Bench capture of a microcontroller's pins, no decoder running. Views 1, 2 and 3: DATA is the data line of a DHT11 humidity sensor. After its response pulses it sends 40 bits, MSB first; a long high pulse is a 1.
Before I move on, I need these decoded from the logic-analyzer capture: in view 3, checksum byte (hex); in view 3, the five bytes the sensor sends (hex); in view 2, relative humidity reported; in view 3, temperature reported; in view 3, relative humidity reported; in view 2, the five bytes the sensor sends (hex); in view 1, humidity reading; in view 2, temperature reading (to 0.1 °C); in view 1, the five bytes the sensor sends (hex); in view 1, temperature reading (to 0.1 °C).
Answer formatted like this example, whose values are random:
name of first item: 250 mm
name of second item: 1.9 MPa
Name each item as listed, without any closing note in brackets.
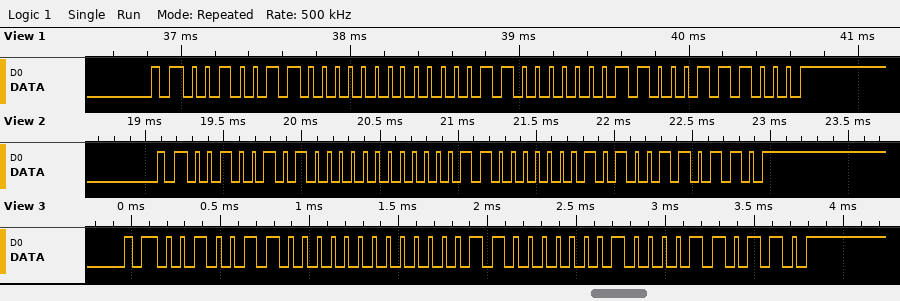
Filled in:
in view 3, checksum byte: 0x36
in view 3, the five bytes the sensor sends: 26 00 0C 04 36
in view 2, relative humidity reported: 37 %
in view 3, temperature reported: 12.4 °C
in view 3, relative humidity reported: 38 %
in view 2, the five bytes the sensor sends: 25 00 0C 05 36
in view 1, humidity reading: 38 %
in view 2, temperature reading: 12.5 °C
in view 1, the five bytes the sensor sends: 26 00 0C 06 38
in view 1, temperature reading: 12.6 °C
